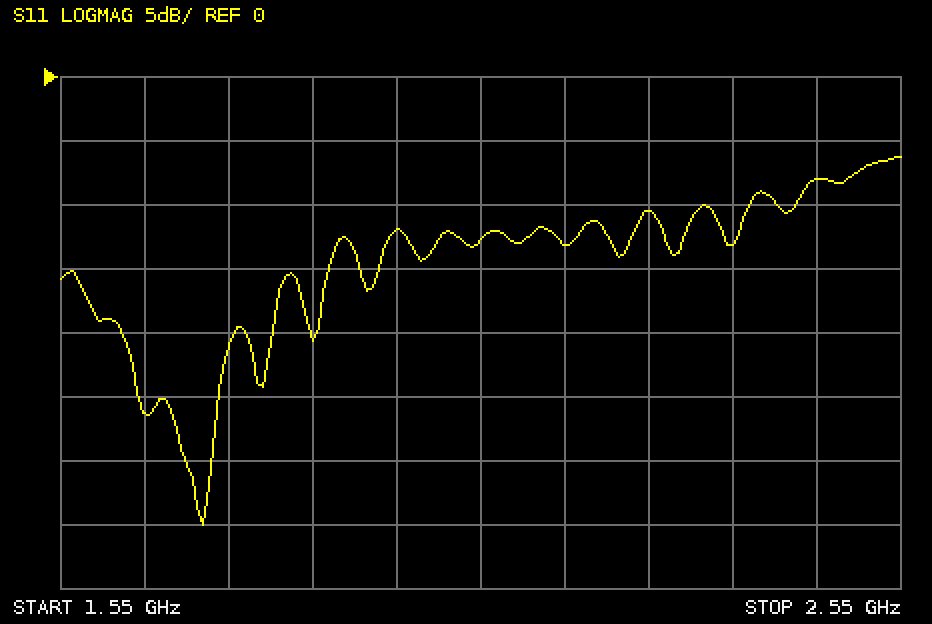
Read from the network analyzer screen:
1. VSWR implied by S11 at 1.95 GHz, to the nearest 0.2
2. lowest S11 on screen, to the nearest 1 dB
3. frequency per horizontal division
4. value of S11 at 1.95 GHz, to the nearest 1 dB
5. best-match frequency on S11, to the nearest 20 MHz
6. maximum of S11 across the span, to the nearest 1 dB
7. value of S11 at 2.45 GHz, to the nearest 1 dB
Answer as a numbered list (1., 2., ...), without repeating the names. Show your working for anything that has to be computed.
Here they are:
1. |Γ| = 10^(-12/20) = 0.2512; VSWR = (1 + 0.2512)/(1 − 0.2512) ≈ 1.67, so 1.6 to the nearest 0.2
2. -35 dB
3. 100 MHz
4. -12 dB
5. 1.72 GHz
6. -6 dB
7. -8 dB
